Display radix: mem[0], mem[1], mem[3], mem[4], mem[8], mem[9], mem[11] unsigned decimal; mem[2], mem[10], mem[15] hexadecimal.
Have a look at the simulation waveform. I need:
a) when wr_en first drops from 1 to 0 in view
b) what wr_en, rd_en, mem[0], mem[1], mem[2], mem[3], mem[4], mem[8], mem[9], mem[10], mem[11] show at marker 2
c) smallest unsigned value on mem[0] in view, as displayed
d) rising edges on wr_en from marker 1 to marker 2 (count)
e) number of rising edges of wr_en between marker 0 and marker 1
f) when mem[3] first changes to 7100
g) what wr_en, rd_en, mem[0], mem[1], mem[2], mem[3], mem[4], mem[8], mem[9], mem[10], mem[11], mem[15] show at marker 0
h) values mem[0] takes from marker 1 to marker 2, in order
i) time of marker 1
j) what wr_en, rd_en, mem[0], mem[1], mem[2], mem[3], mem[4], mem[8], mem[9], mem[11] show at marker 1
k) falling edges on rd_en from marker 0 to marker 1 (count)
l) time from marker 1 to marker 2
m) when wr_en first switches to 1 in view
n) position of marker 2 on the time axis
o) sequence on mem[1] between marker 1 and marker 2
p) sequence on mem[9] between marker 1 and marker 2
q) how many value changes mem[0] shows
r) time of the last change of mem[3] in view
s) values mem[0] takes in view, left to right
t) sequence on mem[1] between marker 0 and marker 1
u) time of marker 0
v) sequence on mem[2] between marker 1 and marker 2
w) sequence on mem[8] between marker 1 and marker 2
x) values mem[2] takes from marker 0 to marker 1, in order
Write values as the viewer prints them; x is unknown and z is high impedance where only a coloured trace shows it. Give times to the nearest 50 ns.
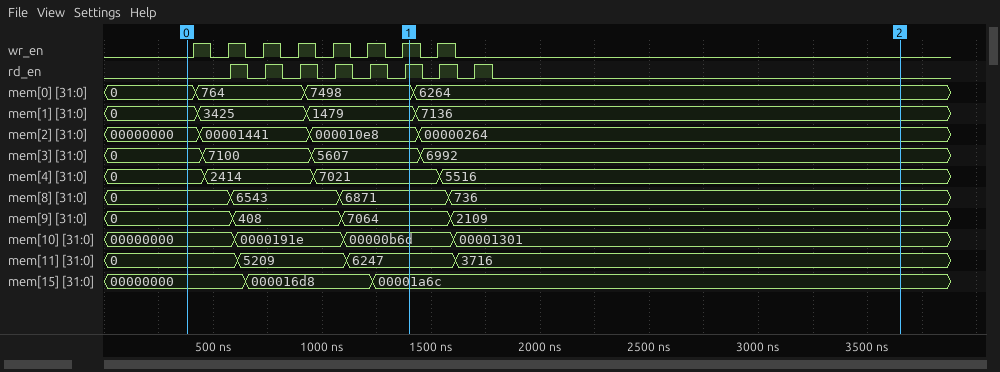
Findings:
500 ns
wr_en=0, rd_en=0, mem[0]=6264, mem[1]=7136, mem[2]=00000264, mem[3]=6992, mem[4]=5516, mem[8]=736, mem[9]=2109, mem[10]=00001301, mem[11]=3716
0
1
7
450 ns
wr_en=0, rd_en=0, mem[0]=0, mem[1]=0, mem[2]=00000000, mem[3]=0, mem[4]=0, mem[8]=0, mem[9]=0, mem[10]=00000000, mem[11]=0, mem[15]=00000000
7498, 6264
1400 ns
wr_en=1, rd_en=1, mem[0]=7498, mem[1]=1479, mem[2]=000010e8, mem[3]=5607, mem[4]=7021, mem[8]=6871, mem[9]=7064, mem[11]=6247
5
2250 ns
400 ns
3650 ns
1479, 7136
7064, 2109
3
1450 ns
0, 764, 7498, 6264
0, 3425, 1479
400 ns
000010e8, 00000264
6871, 736
00000000, 00001441, 000010e8
